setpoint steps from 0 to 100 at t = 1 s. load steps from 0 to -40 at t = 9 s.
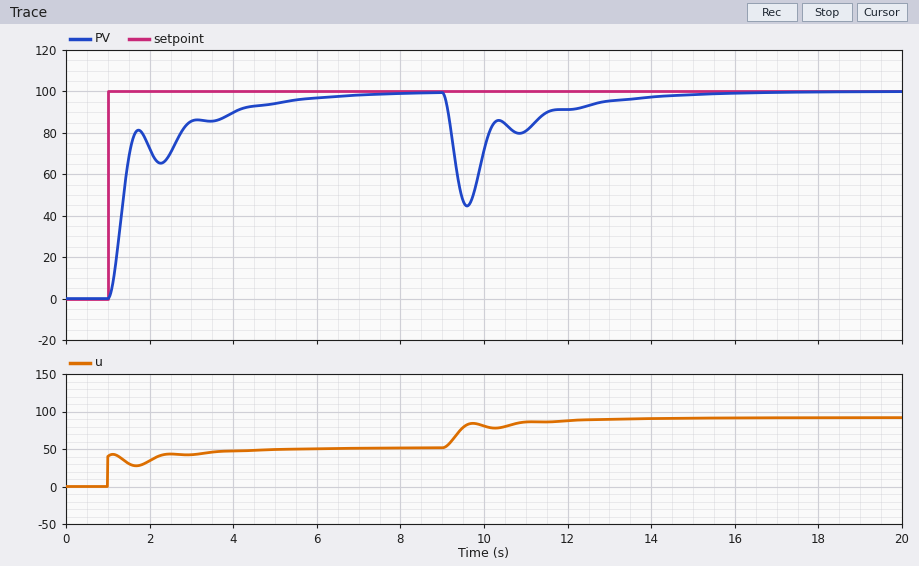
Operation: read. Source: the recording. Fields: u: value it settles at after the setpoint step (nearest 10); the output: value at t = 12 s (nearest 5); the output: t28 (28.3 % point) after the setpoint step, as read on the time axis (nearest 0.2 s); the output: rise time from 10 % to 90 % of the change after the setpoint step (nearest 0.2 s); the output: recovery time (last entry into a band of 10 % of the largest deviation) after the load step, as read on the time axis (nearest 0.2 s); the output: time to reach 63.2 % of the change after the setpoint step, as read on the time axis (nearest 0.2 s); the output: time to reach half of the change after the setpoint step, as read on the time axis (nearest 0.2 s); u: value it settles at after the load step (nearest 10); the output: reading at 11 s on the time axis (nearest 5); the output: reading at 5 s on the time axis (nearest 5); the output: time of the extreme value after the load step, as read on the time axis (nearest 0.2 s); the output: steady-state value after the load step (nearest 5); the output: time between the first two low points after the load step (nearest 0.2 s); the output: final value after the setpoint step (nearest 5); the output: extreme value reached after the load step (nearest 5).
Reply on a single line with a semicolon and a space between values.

50; 90; 1.2 s; 2.8 s; 12.8 s; 1.4 s; 1.4 s; 90; 80; 95; 9.6 s; 100; 1.2 s; 100; 45
